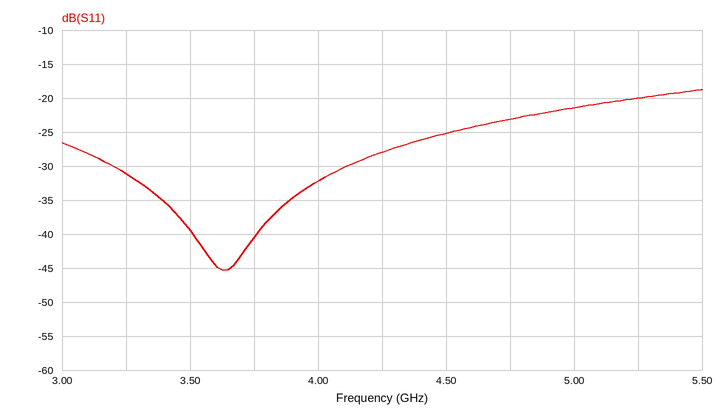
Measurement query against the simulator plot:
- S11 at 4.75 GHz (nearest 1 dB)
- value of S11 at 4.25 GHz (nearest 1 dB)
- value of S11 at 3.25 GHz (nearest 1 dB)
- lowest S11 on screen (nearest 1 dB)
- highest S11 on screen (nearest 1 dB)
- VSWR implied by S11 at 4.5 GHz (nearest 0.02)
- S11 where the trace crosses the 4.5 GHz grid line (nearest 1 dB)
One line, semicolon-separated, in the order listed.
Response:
-23 dB; -28 dB; -31 dB; -45 dB; -19 dB; 1.12; -25 dB
